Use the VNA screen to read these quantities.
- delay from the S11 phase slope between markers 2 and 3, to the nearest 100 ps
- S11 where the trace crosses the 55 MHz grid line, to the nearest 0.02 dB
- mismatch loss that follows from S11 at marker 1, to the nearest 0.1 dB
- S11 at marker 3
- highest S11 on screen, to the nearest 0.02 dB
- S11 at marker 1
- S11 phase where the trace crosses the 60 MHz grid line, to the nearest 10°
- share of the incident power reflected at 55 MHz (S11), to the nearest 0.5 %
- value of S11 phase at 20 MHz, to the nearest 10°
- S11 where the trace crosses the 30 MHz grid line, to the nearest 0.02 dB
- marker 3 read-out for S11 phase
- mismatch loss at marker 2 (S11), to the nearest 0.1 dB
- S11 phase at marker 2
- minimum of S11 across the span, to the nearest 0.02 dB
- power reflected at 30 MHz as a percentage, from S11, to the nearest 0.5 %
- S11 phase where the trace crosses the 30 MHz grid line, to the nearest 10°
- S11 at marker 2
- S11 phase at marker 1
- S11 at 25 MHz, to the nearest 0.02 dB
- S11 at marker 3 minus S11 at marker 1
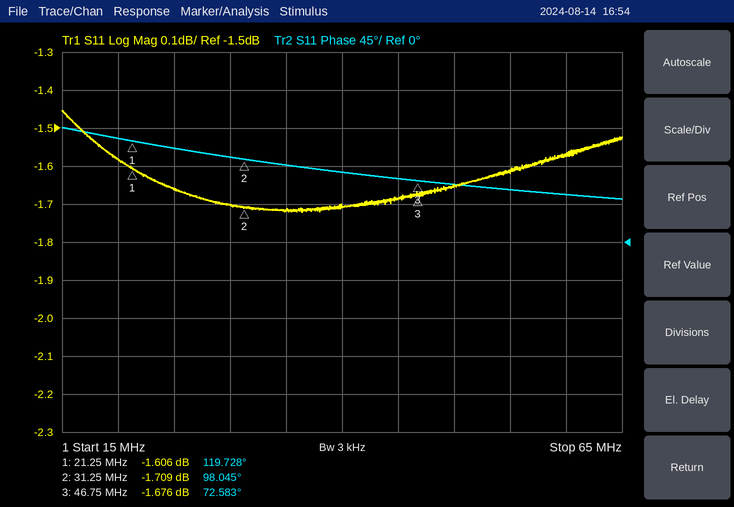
4.6 ns
-1.62 dB
5.1 dB
-1.676 dB
-1.46 dB
-1.606 dB
60°
69.0 %
120°
-1.70 dB
72.583°
4.9 dB
98.045°
-1.72 dB
67.5 %
100°
-1.709 dB
119.728°
-1.66 dB
-0.070 dB
